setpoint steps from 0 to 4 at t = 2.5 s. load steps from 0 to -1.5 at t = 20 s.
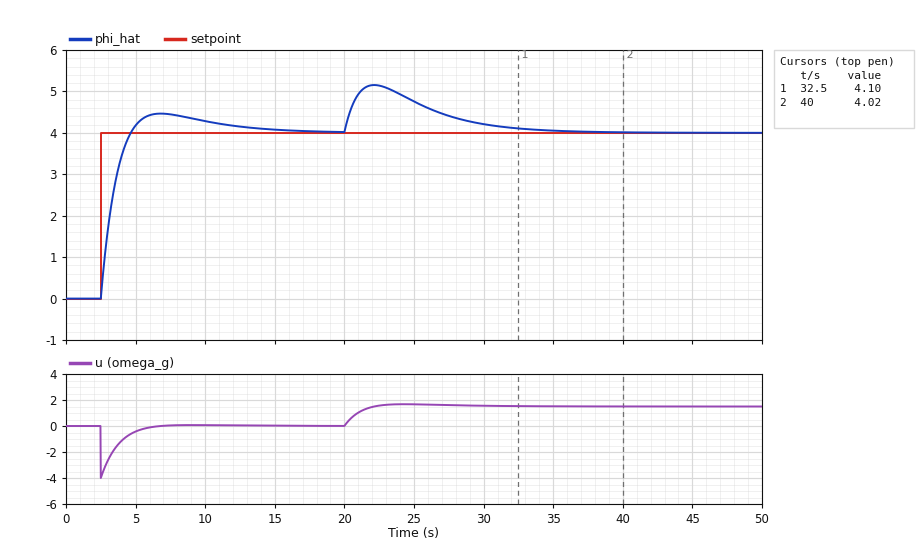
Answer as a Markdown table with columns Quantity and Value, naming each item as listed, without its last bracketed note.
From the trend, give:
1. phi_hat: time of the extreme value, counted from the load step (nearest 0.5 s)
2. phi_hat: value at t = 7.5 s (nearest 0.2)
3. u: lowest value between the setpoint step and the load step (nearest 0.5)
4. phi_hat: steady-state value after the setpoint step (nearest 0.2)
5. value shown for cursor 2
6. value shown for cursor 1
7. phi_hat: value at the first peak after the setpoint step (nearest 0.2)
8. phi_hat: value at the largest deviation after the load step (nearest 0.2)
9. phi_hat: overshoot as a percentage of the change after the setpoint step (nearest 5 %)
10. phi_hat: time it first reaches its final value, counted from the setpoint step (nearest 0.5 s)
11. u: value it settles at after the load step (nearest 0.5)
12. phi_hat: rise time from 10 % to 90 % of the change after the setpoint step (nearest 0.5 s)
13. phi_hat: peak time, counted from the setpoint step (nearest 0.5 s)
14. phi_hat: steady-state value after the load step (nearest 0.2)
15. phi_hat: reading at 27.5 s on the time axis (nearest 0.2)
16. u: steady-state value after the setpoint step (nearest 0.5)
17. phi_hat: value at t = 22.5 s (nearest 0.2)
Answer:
| Quantity | Value |
|---|---|
| phi_hat: time of the extreme value, counted from the load step | 2.0 s |
| phi_hat: value at t = 7.5 s | 4.4 |
| u: lowest value between the setpoint step and the load step | -4.0 |
| phi_hat: steady-state value after the setpoint step | 4.0 |
| value shown for cursor 2 | 4.02 |
| value shown for cursor 1 | 4.10 |
| phi_hat: value at the first peak after the setpoint step | 4.4 |
| phi_hat: value at the largest deviation after the load step | 5.2 |
| phi_hat: overshoot as a percentage of the change after the setpoint step | 10 % |
| phi_hat: time it first reaches its final value, counted from the setpoint step | 2.0 s |
| u: value it settles at after the load step | 1.5 |
| phi_hat: rise time from 10 % to 90 % of the change after the setpoint step | 1.5 s |
| phi_hat: peak time, counted from the setpoint step | 4.5 s |
| phi_hat: steady-state value after the load step | 4.0 |
| phi_hat: reading at 27.5 s on the time axis | 4.4 |
| u: steady-state value after the setpoint step | 0.0 |
| phi_hat: value at t = 22.5 s | 5.2 |
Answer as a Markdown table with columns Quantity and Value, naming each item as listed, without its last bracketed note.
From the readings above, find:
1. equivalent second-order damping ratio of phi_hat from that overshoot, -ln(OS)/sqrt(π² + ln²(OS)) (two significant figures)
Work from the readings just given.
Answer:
| Quantity | Value |
|---|---|
| equivalent second-order damping ratio of phi_hat from that overshoot, -ln(OS)/sqrt(π² + ln²(OS)) | 0.59 |
